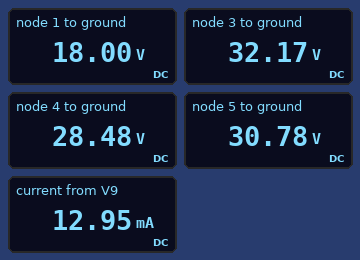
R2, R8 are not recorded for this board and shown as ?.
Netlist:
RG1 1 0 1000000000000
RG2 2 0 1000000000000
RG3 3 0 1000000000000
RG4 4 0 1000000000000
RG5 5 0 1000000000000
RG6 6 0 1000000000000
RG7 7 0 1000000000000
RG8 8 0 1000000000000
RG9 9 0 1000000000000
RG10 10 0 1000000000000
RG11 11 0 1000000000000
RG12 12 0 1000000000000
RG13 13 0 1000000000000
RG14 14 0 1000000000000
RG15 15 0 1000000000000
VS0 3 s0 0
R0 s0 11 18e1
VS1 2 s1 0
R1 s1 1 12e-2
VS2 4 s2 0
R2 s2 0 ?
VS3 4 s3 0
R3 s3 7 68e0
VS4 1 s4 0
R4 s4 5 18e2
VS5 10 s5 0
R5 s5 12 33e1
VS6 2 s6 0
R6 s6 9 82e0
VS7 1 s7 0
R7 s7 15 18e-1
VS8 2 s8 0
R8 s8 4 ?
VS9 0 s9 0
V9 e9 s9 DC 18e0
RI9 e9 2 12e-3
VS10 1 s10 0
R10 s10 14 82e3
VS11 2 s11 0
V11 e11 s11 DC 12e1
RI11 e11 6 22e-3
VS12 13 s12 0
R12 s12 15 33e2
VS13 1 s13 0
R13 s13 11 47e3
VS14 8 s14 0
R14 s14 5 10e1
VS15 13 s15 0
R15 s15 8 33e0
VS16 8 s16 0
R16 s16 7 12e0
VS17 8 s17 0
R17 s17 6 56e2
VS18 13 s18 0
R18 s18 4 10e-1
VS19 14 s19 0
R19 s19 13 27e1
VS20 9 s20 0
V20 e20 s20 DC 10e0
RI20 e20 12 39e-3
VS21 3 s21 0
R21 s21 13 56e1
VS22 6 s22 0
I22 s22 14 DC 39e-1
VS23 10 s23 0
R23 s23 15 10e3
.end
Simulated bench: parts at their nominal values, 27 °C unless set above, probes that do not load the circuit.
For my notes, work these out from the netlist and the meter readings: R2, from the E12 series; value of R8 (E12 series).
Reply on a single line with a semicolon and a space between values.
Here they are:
2.2 kΩ; 2.7 Ω
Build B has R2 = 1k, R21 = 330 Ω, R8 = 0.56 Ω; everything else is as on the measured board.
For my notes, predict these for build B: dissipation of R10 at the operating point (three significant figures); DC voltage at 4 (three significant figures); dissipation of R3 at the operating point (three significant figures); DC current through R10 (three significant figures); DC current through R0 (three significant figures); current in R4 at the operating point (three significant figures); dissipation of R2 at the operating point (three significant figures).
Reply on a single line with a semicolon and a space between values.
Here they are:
13.6 W; 20.2 V; 105 mW; 12.9 mA; 127 µA; 2.80 mA; 407 mW
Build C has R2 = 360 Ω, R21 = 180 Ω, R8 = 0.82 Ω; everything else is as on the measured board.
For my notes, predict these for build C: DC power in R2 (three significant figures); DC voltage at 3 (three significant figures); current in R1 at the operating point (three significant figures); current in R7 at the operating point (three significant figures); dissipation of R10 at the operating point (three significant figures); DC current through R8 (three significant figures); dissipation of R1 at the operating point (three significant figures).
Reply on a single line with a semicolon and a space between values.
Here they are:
1.24 W; 25.0 V; 19.4 mA; 3.08 mA; 13.6 W; 3.84 A; 45.3 µW
